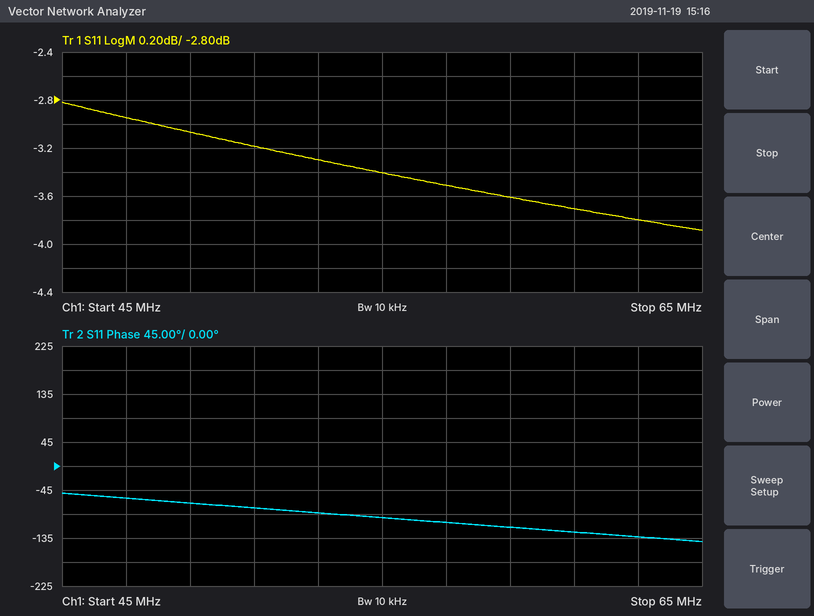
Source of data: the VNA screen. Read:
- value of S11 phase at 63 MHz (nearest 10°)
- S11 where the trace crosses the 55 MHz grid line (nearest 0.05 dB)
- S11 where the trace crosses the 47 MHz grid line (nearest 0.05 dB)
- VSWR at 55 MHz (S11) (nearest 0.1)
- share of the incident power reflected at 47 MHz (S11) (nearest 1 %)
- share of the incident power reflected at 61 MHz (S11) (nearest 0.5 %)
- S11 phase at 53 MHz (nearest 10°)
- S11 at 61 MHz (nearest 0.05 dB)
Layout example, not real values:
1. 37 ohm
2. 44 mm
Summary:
1. -130°
2. -3.40 dB
3. -2.95 dB
4. 5.2
5. 51 %
6. 42.5 %
7. -90°
8. -3.70 dB
